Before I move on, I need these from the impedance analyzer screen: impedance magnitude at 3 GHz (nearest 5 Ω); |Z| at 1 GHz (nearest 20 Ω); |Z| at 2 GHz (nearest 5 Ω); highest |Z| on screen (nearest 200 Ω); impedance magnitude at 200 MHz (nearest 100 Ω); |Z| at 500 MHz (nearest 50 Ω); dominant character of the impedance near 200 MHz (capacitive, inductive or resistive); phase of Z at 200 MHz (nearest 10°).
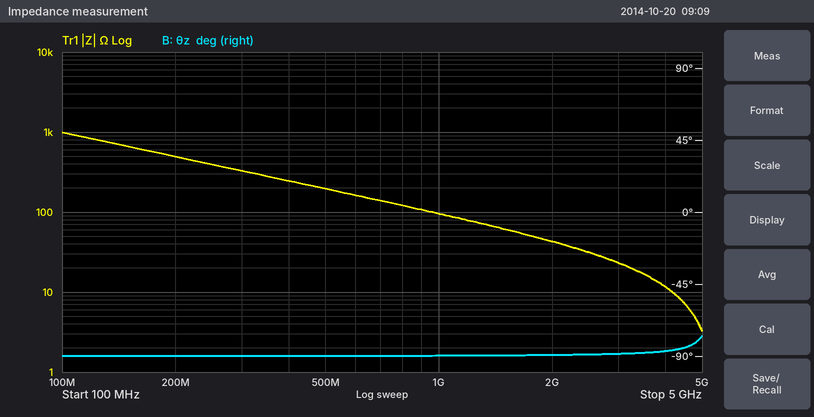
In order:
25 Ω
100 Ω
45 Ω
1.0 kΩ
500 Ω
200 Ω
capacitive
-90°
